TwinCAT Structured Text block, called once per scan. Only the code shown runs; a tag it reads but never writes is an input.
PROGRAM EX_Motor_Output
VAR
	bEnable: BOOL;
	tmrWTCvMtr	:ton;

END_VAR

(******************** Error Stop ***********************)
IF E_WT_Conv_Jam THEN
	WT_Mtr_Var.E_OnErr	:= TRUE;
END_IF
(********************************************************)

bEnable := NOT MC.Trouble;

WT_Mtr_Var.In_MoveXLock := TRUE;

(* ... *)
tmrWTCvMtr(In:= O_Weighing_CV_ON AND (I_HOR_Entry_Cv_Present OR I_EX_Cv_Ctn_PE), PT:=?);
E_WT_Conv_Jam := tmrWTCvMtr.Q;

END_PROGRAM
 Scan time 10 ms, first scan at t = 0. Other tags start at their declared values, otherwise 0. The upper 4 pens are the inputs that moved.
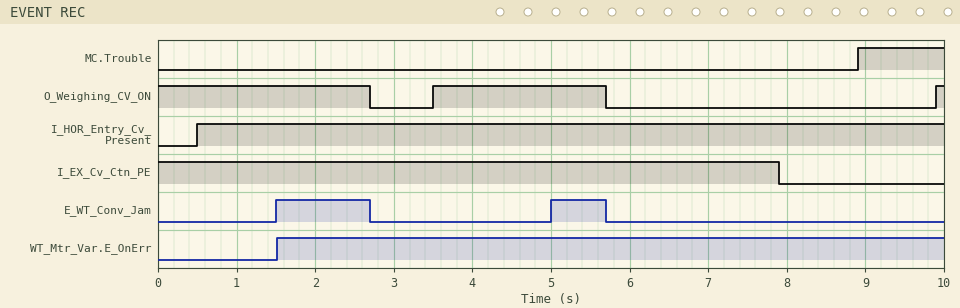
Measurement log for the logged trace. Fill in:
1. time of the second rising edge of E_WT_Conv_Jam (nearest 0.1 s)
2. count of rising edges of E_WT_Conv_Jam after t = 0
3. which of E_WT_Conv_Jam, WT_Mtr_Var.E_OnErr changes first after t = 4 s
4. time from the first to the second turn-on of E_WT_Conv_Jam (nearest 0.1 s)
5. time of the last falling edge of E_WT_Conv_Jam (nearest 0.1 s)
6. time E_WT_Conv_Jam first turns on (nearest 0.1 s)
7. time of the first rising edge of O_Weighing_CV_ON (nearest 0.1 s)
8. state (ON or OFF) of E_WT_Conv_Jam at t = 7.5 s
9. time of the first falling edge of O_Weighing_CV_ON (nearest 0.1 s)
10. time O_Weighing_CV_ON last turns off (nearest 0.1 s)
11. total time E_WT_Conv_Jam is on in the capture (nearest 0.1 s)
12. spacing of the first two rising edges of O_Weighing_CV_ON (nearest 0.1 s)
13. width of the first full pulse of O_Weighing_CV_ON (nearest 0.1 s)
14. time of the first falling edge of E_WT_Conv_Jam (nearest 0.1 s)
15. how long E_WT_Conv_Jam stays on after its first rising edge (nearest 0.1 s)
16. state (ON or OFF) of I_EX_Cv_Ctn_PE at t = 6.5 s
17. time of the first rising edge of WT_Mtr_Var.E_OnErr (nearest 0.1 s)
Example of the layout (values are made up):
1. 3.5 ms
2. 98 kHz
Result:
1. 5.0 s
2. 2
3. E_WT_Conv_Jam
4. 3.5 s
5. 5.7 s
6. 1.5 s
7. 3.5 s
8. OFF
9. 2.7 s
10. 5.7 s
11. 1.9 s
12. 6.4 s
13. 2.2 s
14. 2.7 s
15. 1.2 s
16. ON
17. 1.5 s
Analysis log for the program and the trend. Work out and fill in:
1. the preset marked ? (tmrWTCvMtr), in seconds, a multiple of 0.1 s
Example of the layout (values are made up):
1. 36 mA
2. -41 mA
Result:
1. 1.5 s
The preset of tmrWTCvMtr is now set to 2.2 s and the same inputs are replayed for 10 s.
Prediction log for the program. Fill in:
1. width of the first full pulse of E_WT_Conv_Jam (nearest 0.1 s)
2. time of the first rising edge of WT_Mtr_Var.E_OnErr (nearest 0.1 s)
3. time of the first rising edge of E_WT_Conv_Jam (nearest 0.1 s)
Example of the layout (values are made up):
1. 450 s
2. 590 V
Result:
1. 0.5 s
2. 2.2 s
3. 2.2 s
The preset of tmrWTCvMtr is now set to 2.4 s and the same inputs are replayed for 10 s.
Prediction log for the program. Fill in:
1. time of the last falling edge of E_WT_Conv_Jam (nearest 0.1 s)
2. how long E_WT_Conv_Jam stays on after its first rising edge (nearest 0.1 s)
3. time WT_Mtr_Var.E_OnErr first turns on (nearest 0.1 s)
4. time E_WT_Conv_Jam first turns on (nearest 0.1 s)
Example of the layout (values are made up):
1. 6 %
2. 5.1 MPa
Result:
1. 2.7 s
2. 0.3 s
3. 2.4 s
4. 2.4 s
